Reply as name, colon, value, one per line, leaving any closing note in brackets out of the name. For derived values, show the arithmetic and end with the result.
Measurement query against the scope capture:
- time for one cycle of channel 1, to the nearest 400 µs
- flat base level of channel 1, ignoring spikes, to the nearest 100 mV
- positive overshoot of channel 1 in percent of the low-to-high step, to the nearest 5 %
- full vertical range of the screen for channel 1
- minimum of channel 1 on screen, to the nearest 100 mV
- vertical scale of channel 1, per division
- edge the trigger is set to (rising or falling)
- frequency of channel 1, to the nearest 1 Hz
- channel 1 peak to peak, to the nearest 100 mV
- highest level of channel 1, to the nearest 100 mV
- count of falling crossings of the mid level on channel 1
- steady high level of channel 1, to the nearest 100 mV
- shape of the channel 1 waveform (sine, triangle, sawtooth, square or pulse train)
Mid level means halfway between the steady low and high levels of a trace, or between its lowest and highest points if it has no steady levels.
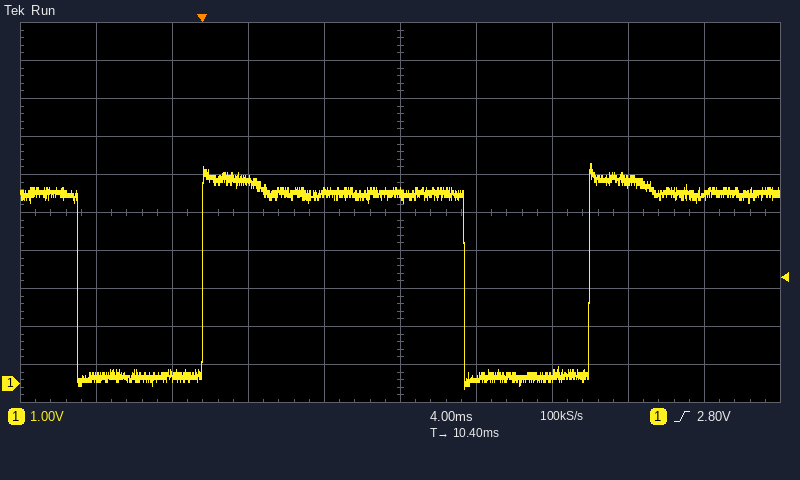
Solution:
time for one cycle of channel 1, to the nearest 400 µs: 20.4 ms
flat base level of channel 1, ignoring spikes, to the nearest 100 mV: 200 mV
positive overshoot of channel 1 in percent of the low-to-high step, to the nearest 5 %: 15 %
full vertical range of the screen for channel 1: 10 V
minimum of channel 1 on screen, to the nearest 100 mV: -100 mV
vertical scale of channel 1, per division: 1 V
edge the trigger is set to: rising
frequency of channel 1, to the nearest 1 Hz: 1 / 20.4 ms ≈ 49 Hz
channel 1 peak to peak, to the nearest 100 mV: 5.8 V − (-100 mV) = 5.9 V
highest level of channel 1, to the nearest 100 mV: 5.8 V
count of falling crossings of the mid level on channel 1: 2
steady high level of channel 1, to the nearest 100 mV: 5.0 V
shape of the channel 1 waveform: pulse train
